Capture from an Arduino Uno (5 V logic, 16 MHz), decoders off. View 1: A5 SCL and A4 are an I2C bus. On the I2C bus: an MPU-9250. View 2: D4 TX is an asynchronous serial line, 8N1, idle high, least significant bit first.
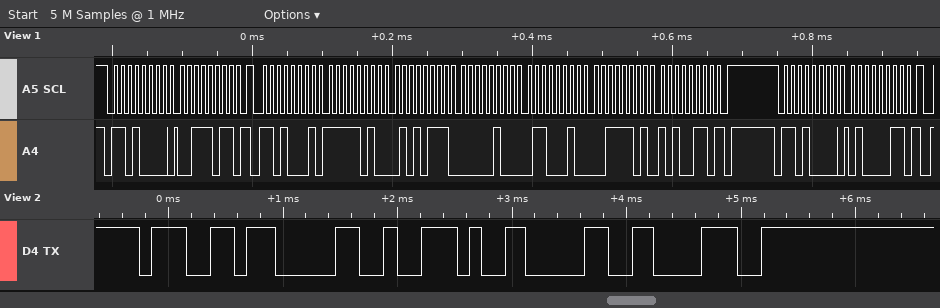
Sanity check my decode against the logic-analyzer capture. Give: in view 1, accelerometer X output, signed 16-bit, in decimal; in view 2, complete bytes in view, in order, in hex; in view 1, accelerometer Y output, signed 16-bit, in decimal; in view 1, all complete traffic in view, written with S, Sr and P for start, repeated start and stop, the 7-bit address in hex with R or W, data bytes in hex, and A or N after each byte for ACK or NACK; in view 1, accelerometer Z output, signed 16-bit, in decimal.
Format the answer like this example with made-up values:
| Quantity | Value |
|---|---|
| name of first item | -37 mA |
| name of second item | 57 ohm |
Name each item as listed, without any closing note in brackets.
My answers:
| Quantity | Value |
|---|---|
| in view 1, accelerometer X output, signed 16-bit, in decimal | -1449 |
| in view 2, complete bytes in view, in order, in hex | 67 30 2E 30 38 |
| in view 1, accelerometer Y output, signed 16-bit, in decimal | 1122 |
| in view 1, all complete traffic in view, written with S, Sr and P for start, repeated start and stop, the 7-bit address in hex with R or W, data bytes in hex, and A or N after each byte for ACK or NACK | S 68W A 3B A Sr 68R A FA A 57 A 04 A 62 A 3D A A6 N P S 68W A 43 A |
| in view 1, accelerometer Z output, signed 16-bit, in decimal | 15782 |
